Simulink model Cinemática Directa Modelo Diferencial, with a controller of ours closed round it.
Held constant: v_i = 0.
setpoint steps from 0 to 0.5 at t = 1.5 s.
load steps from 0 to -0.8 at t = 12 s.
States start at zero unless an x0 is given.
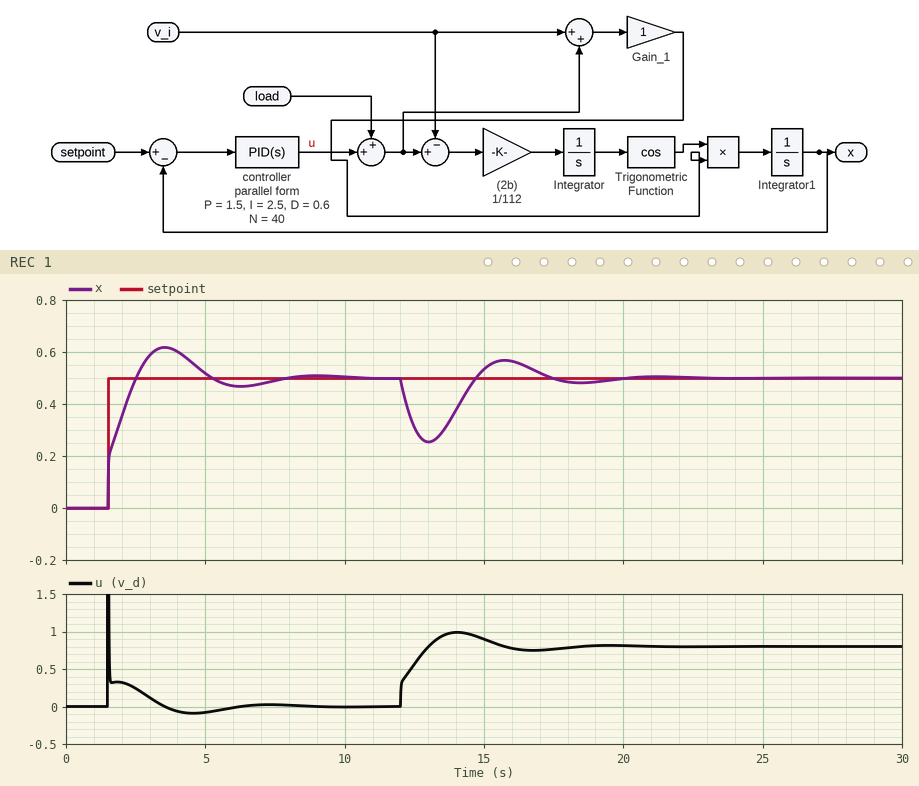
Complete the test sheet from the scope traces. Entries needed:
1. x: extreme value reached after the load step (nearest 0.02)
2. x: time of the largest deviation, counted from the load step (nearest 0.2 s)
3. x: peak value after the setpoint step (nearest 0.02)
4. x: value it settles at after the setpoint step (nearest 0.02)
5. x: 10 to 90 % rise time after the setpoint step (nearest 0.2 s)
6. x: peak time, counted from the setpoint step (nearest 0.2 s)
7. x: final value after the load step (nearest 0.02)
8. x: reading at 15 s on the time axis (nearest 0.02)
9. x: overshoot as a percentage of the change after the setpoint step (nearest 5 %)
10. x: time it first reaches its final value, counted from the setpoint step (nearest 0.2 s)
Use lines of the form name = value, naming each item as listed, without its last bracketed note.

x: extreme value reached after the load step = 0.26
x: time of the largest deviation, counted from the load step = 1.0 s
x: peak value after the setpoint step = 0.62
x: value it settles at after the setpoint step = 0.50
x: 10 to 90 % rise time after the setpoint step = 0.8 s
x: peak time, counted from the setpoint step = 2.0 s
x: final value after the load step = 0.50
x: reading at 15 s on the time axis = 0.54
x: overshoot as a percentage of the change after the setpoint step = 25 %
x: time it first reaches its final value, counted from the setpoint step = 1.0 s
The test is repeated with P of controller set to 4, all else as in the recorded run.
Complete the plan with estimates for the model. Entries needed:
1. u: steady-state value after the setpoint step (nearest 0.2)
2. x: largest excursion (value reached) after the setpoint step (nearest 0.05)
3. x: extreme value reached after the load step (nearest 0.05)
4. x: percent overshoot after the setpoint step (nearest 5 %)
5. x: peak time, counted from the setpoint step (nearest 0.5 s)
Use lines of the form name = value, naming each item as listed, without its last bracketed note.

u: steady-state value after the setpoint step = 0.0
x: largest excursion (value reached) after the setpoint step = 0.55
x: extreme value reached after the load step = 0.35
x: percent overshoot after the setpoint step = 10 %
x: peak time, counted from the setpoint step = 1.5 s
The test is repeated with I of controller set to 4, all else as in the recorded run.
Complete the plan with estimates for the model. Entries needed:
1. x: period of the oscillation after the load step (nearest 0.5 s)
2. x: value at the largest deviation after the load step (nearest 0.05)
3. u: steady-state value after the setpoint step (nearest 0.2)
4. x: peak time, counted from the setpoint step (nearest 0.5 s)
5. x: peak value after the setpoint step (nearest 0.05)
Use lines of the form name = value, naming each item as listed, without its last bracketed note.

x: period of the oscillation after the load step = 4.0 s
x: value at the largest deviation after the load step = 0.30
u: steady-state value after the setpoint step = 0.0
x: peak time, counted from the setpoint step = 1.5 s
x: peak value after the setpoint step = 0.65
